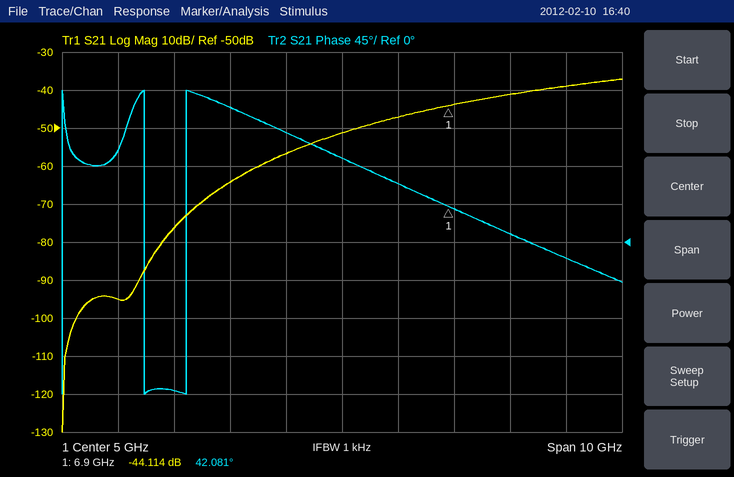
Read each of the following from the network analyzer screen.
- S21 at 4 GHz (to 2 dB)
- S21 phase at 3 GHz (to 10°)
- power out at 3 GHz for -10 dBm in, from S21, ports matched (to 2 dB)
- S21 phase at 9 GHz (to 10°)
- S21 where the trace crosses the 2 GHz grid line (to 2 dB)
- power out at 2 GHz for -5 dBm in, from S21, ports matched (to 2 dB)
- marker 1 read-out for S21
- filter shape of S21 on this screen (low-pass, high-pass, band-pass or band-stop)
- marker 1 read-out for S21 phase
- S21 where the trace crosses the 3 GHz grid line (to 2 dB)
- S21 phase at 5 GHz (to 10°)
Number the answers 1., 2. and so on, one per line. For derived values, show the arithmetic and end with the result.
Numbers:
1. -56 dB
2. 160°
3. -10 dBm + (-64 dB) = -74 dBm
4. -20°
5. -76 dB
6. -5 dBm + (-76 dB) = -82 dBm
7. -44.114 dB
8. high-pass
9. 42.081°
10. -64 dB
11. 100°
